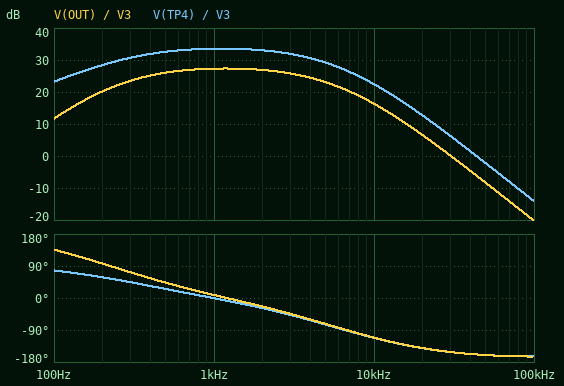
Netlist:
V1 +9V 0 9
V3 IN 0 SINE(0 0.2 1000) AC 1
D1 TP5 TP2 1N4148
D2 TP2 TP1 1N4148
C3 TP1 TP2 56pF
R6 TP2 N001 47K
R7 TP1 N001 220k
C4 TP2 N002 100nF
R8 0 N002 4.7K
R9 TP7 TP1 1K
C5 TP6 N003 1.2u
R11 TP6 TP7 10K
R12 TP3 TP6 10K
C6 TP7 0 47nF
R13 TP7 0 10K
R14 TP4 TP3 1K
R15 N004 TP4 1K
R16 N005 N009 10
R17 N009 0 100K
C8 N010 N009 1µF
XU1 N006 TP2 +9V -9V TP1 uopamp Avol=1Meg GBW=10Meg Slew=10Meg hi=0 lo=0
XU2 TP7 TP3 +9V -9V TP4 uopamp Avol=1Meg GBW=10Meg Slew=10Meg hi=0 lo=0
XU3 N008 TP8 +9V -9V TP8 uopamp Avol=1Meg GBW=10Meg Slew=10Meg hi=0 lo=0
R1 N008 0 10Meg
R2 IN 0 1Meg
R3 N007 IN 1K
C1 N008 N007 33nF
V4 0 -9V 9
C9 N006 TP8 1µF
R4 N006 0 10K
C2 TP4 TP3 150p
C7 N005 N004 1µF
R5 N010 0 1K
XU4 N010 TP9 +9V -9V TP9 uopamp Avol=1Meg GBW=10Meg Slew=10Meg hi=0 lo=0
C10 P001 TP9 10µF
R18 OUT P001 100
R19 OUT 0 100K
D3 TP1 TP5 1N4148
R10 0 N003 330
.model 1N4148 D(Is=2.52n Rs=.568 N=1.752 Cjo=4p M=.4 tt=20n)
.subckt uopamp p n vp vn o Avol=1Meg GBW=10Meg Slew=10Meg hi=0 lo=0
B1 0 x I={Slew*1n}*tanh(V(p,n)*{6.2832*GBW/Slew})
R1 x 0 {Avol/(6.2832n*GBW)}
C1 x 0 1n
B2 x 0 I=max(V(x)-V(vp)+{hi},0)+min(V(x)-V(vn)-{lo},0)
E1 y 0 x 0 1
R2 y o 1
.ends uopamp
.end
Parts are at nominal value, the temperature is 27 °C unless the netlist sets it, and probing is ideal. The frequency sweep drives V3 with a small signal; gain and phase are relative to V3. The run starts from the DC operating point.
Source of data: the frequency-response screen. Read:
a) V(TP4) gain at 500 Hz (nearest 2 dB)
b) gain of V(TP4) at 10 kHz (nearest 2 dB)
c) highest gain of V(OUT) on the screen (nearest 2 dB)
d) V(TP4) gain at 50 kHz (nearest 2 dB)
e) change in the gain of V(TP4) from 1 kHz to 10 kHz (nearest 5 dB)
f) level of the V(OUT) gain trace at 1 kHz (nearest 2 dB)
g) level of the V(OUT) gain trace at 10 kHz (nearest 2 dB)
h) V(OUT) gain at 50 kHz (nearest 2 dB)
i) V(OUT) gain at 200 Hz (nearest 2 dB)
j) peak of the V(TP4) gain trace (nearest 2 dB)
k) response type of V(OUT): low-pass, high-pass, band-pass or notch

32 dB
22 dB
28 dB
-2 dB
-10 dB
28 dB
16 dB
-8 dB
20 dB
34 dB
band-pass
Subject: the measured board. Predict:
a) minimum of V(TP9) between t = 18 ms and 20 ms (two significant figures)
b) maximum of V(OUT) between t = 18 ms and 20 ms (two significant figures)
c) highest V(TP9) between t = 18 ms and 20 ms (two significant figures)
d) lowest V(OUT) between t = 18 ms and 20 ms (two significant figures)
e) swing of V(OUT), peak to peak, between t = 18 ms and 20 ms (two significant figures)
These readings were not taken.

-370 mV
390 mV
390 mV
-370 mV
750 mV
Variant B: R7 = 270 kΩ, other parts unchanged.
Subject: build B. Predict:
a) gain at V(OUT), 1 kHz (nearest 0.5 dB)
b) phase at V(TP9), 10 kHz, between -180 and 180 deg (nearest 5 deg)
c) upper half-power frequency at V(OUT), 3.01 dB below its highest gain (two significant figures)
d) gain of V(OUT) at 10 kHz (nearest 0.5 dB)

28.5 dB
-115 deg
3.9 kHz
17.0 dB
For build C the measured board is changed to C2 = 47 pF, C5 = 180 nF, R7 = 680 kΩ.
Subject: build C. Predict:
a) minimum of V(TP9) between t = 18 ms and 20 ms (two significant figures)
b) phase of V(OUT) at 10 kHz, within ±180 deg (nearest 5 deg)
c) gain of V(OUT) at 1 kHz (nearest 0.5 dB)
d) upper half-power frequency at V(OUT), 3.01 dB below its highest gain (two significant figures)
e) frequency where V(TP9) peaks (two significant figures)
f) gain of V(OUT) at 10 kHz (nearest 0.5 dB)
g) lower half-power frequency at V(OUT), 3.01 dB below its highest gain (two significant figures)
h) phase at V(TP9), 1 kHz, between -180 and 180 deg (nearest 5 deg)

-370 mV
-135 deg
35.5 dB
2.9 kHz
990 Hz
18.5 dB
330 Hz
0 deg
